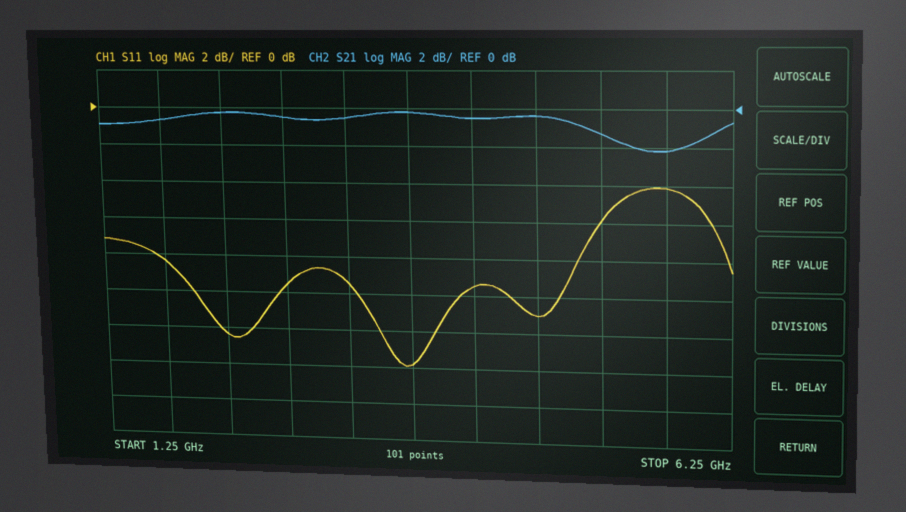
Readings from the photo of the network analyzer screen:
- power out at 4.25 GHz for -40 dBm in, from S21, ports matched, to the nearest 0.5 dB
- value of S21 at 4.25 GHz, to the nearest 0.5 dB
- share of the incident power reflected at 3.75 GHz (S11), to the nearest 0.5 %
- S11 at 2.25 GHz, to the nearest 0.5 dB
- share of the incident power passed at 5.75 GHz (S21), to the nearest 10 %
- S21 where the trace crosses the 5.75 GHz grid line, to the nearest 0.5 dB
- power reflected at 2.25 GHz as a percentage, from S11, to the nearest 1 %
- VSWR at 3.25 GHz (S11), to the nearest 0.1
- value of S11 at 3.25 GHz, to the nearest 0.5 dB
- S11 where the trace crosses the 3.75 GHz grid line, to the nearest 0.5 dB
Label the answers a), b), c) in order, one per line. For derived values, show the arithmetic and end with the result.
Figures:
a) -40 dBm + (-0.5 dB) = -40.5 dBm
b) -0.5 dB
c) 10^(-14/10) ≈ 4.0 %
d) -12.5 dB
e) 10^(-2/10) ≈ 63.1 %, so 60 % to the nearest 10 %
f) -2.0 dB
g) 10^(-12.5/10) ≈ 6 %
h) |Γ| = 10^(-9.5/20) = 0.3350; VSWR = (1 + 0.3350)/(1 − 0.3350) ≈ 2.0
i) -9.5 dB
j) -14.0 dB
